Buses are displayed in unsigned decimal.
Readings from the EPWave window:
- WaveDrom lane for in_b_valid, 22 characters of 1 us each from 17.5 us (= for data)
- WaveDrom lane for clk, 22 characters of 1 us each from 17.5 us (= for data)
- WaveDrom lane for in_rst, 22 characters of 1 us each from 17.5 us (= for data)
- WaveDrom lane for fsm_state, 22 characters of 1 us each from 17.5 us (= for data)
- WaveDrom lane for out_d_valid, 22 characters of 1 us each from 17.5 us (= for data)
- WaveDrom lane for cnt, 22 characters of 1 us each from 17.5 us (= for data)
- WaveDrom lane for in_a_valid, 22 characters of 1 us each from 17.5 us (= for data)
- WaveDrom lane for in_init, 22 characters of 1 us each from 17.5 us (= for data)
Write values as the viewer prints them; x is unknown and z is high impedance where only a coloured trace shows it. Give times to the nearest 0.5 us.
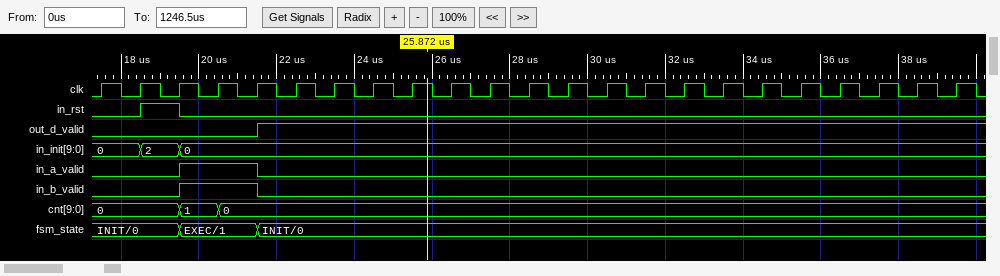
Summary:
{name: 'in_b_valid', wave: '0.1.0.................'}
{name: 'clk', wave: 'p.....................'}
{name: 'in_rst', wave: '010...................'}
{name: 'fsm_state', wave: '=.=.=.................', data: 'INIT/0 EXEC/1 INIT/0'}
{name: 'out_d_valid', wave: '0...1.................'}
{name: 'cnt', wave: '=.==..................', data: '0 1 0'}
{name: 'in_a_valid', wave: '0.1.0.................'}
{name: 'in_init', wave: '===...................', data: '0 2 0'}
